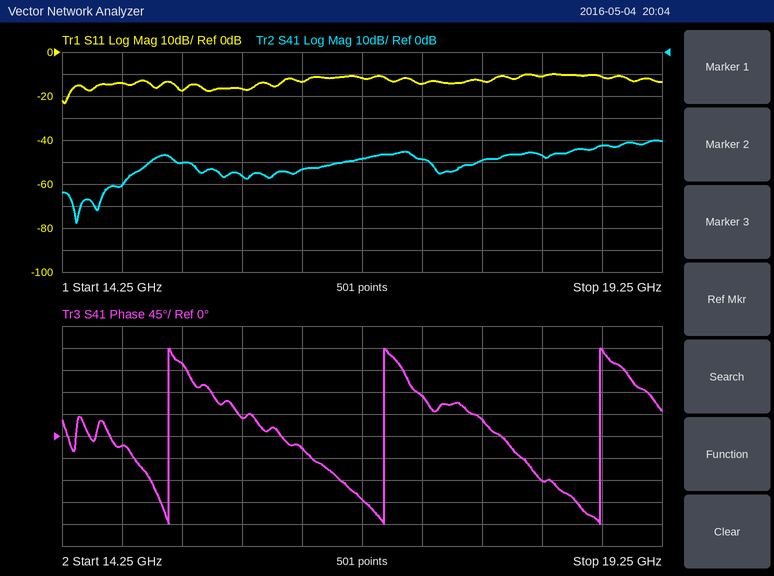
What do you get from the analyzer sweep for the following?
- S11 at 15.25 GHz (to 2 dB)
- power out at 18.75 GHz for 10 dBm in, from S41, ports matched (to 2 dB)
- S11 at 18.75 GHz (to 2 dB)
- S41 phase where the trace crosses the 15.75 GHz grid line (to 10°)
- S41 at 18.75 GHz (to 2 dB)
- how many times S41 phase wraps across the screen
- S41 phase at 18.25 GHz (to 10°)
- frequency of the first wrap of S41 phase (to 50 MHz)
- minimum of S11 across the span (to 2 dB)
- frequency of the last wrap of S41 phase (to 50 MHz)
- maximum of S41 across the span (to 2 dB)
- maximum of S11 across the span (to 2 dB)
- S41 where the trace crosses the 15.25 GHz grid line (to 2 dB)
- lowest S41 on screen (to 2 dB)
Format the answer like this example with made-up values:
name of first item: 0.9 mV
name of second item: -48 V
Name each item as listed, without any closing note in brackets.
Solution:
S11 at 15.25 GHz: -18 dB
power out at 18.75 GHz for 10 dBm in, from S41, ports matched: -32 dBm
S11 at 18.75 GHz: -12 dB
S41 phase where the trace crosses the 15.75 GHz grid line: 40°
S41 at 18.75 GHz: -42 dB
how many times S41 phase wraps across the screen: 3
S41 phase at 18.25 GHz: -90°
frequency of the first wrap of S41 phase: 15.15 GHz
minimum of S11 across the span: -24 dB
frequency of the last wrap of S41 phase: 18.75 GHz
maximum of S41 across the span: -40 dB
maximum of S11 across the span: -10 dB
S41 where the trace crosses the 15.25 GHz grid line: -50 dB
lowest S41 on screen: -78 dB
